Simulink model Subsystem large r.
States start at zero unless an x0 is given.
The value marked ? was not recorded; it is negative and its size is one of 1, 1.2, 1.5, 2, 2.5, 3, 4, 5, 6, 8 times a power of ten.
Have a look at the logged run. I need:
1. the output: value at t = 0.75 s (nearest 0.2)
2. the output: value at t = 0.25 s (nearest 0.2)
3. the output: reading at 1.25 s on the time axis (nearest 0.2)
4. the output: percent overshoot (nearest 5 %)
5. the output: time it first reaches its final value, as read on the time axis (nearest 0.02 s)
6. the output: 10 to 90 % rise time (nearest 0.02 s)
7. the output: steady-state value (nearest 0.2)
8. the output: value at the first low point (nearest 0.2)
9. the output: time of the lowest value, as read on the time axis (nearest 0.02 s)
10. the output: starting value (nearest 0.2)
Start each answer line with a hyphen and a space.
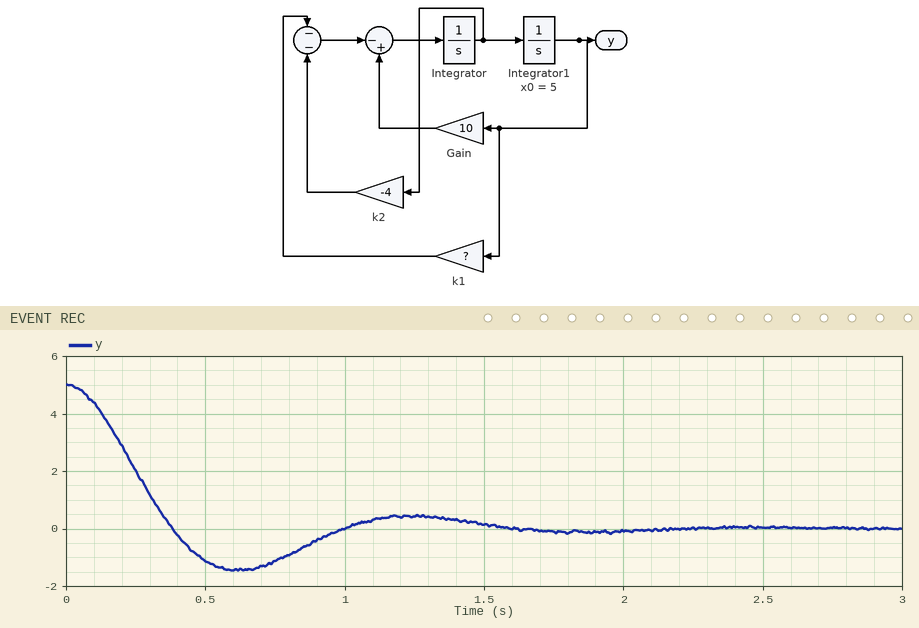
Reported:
- -1.2
- 2.0
- 0.4
- 30 %
- 0.38 s
- 0.26 s
- 0.0
- -1.4
- 0.62 s
- 5.0
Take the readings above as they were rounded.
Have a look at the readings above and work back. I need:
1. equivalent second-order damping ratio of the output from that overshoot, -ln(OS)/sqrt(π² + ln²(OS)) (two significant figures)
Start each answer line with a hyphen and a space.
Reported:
- 0.36
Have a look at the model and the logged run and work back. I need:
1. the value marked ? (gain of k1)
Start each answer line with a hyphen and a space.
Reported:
- -40
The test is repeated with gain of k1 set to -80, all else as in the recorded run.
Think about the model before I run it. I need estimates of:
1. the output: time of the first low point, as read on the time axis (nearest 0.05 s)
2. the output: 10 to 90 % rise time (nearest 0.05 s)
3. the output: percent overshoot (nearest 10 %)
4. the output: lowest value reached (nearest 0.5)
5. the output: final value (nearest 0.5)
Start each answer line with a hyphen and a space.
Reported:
- 0.40 s
- 0.15 s
- 50 %
- -2.5
- 0.0
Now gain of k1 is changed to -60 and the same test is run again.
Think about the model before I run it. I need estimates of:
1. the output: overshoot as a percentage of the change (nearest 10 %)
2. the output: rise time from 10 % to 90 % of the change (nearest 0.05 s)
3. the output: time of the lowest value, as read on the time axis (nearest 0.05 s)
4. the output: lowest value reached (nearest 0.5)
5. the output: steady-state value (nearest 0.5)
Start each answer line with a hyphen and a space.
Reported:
- 40 %
- 0.20 s
- 0.45 s
- -2.0
- 0.0
